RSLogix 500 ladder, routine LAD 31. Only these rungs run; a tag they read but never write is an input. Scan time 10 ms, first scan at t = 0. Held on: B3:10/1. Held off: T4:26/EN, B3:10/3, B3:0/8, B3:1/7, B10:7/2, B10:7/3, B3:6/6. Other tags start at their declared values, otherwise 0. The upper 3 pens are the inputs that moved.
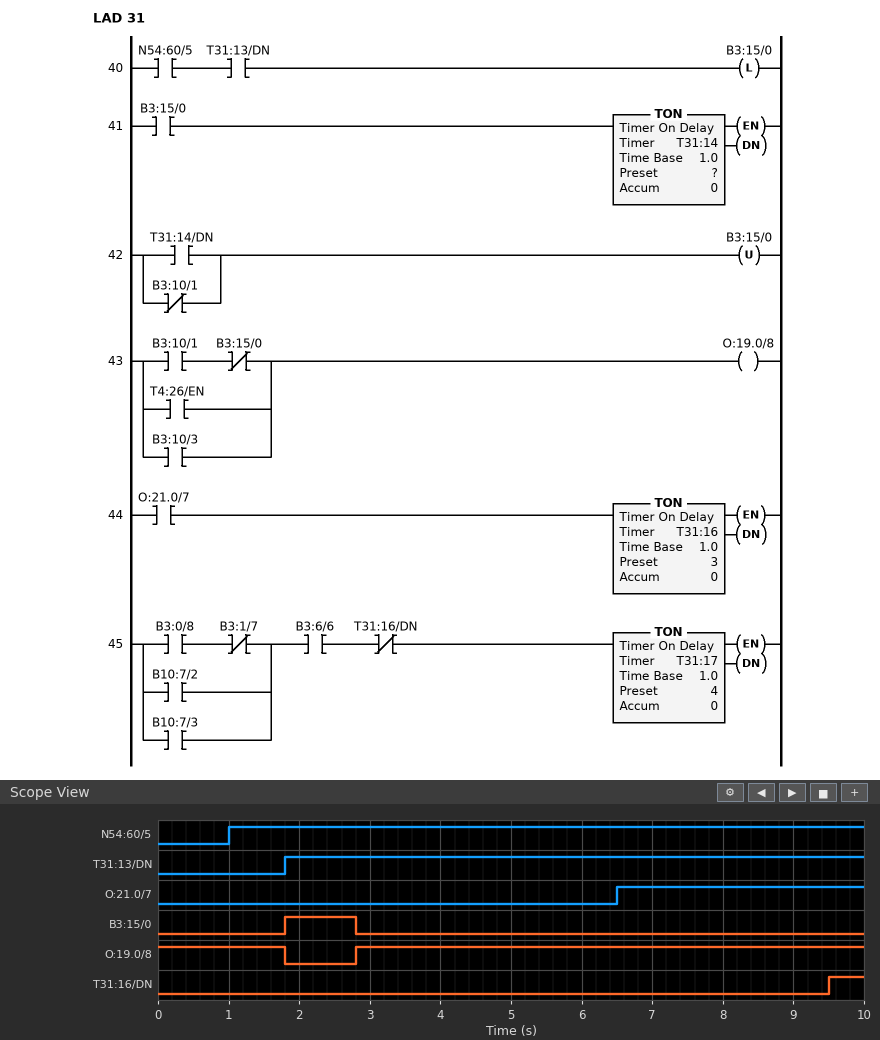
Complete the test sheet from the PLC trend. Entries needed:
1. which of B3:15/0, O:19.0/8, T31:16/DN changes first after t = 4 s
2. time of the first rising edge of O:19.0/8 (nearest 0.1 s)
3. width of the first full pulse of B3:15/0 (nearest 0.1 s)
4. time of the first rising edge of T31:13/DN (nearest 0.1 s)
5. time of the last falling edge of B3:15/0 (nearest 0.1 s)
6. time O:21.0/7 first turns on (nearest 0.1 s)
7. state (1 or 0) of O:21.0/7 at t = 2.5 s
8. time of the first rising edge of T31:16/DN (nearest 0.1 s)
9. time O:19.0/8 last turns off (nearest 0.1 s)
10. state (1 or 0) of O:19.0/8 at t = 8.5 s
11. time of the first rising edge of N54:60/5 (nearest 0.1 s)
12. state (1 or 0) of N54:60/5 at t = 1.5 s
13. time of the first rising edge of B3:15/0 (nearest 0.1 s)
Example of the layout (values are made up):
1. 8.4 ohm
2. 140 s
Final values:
1. T31:16/DN
2. 2.8 s
3. 1.0 s
4. 1.8 s
5. 2.8 s
6. 6.5 s
7. 0
8. 9.5 s
9. 1.8 s
10. 1
11. 1.0 s
12. 1
13. 1.8 s
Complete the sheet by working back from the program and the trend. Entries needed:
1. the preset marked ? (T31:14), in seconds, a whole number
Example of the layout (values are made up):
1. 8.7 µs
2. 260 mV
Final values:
1. 1 s
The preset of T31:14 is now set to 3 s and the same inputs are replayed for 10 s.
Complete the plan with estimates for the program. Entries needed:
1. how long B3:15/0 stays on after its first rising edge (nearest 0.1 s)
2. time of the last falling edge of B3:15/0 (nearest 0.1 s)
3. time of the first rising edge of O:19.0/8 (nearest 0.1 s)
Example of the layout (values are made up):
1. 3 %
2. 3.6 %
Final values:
1. 3.0 s
2. 4.8 s
3. 4.8 s
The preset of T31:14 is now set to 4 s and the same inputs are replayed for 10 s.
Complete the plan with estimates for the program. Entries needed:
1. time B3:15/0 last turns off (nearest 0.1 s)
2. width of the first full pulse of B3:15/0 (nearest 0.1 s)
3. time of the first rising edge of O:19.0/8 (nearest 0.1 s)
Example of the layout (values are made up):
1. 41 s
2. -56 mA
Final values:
1. 5.8 s
2. 4.0 s
3. 5.8 s
